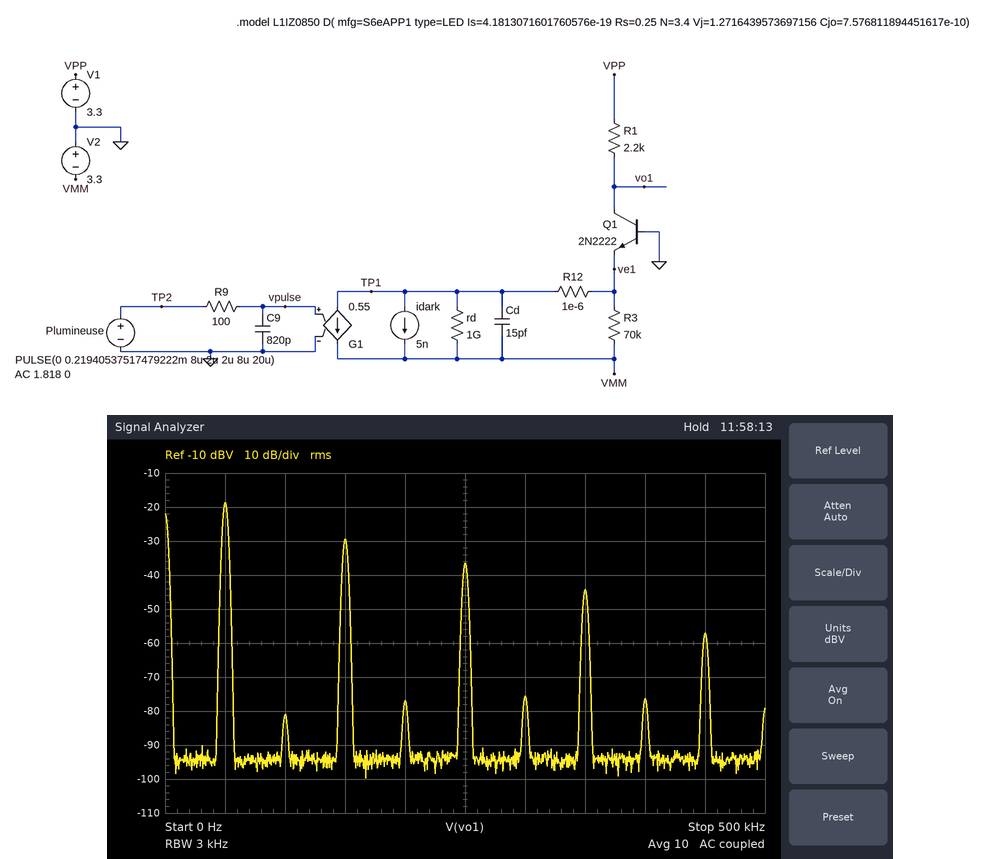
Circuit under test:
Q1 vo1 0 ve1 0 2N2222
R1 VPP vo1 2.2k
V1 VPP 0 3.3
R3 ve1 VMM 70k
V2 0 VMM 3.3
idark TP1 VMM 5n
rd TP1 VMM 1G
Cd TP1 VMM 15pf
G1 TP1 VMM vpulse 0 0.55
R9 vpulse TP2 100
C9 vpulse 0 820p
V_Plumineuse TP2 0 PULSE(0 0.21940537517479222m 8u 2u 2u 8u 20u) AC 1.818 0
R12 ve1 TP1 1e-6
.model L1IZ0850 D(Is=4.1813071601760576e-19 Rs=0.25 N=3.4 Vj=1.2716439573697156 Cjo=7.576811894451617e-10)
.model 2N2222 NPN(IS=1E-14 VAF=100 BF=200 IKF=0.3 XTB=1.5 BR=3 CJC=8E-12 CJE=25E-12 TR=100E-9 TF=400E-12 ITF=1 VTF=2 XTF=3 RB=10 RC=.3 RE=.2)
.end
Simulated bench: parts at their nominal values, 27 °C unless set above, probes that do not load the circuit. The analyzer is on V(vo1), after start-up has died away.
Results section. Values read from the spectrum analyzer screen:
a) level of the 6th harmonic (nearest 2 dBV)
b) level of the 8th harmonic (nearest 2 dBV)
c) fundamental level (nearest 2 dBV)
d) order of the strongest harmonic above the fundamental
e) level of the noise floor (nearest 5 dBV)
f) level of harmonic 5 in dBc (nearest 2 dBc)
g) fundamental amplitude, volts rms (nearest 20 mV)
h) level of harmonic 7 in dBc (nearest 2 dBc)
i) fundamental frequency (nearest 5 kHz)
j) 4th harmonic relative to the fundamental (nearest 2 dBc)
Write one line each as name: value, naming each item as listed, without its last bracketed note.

level of the 6th harmonic: -76 dBV
level of the 8th harmonic: -76 dBV
fundamental level: -18 dBV
order of the strongest harmonic above the fundamental: 3
level of the noise floor: -95 dBV
level of harmonic 5 in dBc: -18 dBc
fundamental amplitude, volts rms: 120 mV
level of harmonic 7 in dBc: -26 dBc
fundamental frequency: 50 kHz
4th harmonic relative to the fundamental: -58 dBc
